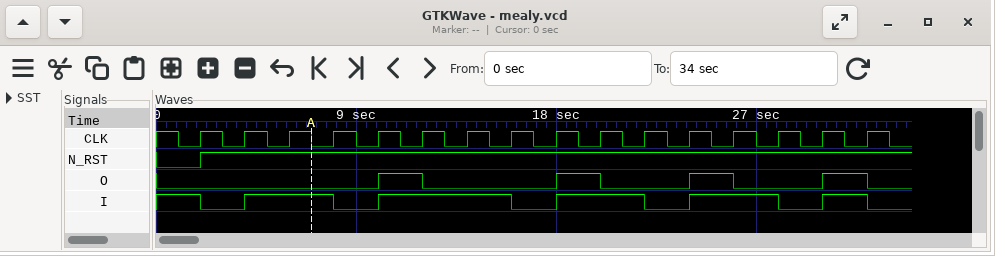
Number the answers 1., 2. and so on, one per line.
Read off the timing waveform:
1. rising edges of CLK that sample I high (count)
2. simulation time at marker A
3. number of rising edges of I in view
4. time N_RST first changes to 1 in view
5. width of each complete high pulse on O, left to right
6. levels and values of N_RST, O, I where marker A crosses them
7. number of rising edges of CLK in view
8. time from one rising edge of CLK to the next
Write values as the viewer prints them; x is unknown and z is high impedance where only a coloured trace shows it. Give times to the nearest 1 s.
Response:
1. 11
2. 7 s
3. 5
4. 2 s
5. 2 s, 2 s, 2 s, 2 s
6. N_RST=1, O=0, I=1
7. 16
8. 2 s
